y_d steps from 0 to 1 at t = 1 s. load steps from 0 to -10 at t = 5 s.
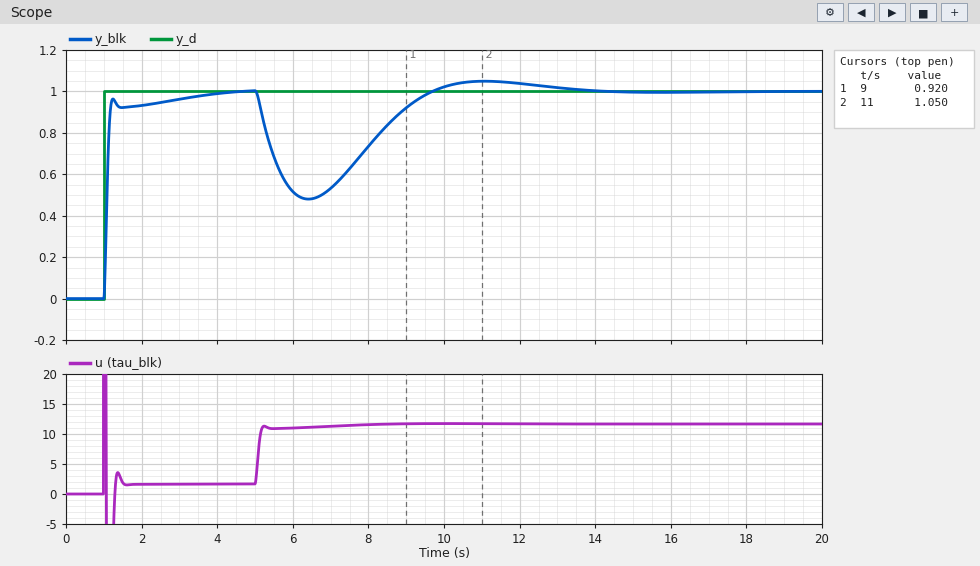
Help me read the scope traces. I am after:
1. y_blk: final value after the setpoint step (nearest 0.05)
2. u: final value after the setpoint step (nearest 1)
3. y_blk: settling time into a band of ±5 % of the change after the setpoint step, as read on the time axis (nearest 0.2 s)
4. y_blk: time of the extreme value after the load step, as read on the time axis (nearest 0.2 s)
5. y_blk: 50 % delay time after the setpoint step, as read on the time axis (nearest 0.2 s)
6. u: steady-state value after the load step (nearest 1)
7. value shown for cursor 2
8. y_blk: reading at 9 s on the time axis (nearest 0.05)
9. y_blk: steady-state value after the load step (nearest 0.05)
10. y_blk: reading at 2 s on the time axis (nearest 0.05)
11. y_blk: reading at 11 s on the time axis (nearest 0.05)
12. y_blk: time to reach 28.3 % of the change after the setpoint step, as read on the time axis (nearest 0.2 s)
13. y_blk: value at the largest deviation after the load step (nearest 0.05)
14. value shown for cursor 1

1.00
2
2.6 s
6.4 s
1.0 s
12
1.050
0.90
1.00
0.95
1.05
1.0 s
0.50
0.920
